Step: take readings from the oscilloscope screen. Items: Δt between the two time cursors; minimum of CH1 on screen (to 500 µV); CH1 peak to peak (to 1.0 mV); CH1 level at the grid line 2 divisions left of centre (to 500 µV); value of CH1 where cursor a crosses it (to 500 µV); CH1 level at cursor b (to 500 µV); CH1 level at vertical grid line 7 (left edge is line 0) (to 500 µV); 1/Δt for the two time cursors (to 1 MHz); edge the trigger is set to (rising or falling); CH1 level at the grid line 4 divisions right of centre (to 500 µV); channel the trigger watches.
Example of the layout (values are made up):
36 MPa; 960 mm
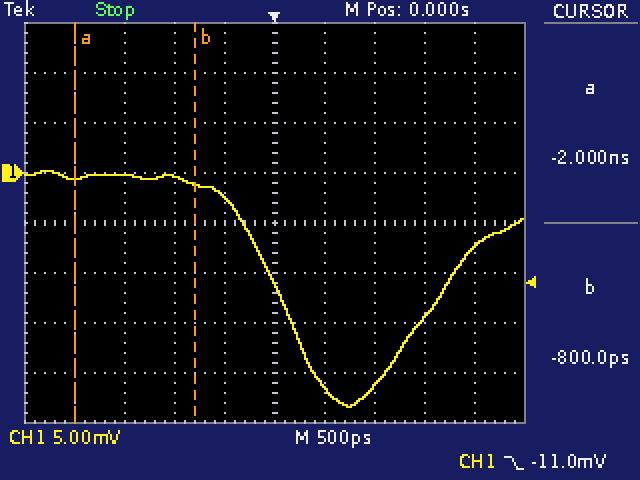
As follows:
1.20 ns; -23.5 mV; 24.0 mV; -500 µV; -500 µV; -1.0 mV; -21.5 mV; 833 MHz; falling; -7.5 mV; CH1
